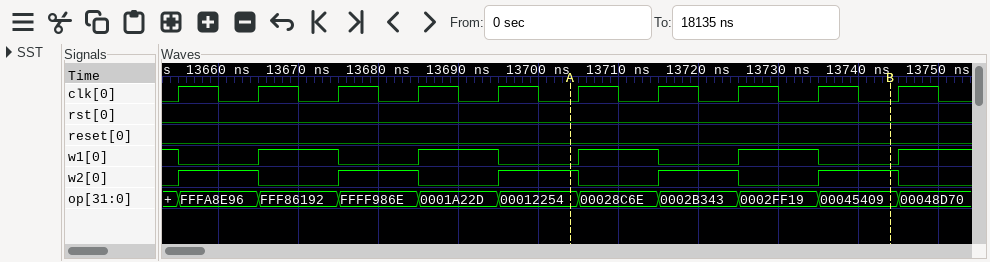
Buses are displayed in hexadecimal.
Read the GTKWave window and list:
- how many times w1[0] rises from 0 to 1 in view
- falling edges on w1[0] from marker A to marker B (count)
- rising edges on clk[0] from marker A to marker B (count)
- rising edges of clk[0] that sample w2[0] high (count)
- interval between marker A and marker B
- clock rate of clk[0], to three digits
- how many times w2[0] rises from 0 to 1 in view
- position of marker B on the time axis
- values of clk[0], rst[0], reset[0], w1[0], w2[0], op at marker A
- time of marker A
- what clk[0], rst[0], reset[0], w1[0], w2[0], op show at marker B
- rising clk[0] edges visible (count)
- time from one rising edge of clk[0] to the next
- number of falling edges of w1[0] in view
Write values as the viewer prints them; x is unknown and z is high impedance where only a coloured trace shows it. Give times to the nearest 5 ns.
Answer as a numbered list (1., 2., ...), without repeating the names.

1. 5
2. 2
3. 4
4. 5
5. 40 ns
6. 100 MHz
7. 5
8. 13745 ns
9. clk[0]=0, rst[0]=0, reset[0]=0, w1[0]=0, w2[0]=1, op=00012254
10. 13705 ns
11. clk[0]=0, rst[0]=0, reset[0]=0, w1[0]=0, w2[0]=1, op=00045409
12. 10
13. 10 ns
14. 5
